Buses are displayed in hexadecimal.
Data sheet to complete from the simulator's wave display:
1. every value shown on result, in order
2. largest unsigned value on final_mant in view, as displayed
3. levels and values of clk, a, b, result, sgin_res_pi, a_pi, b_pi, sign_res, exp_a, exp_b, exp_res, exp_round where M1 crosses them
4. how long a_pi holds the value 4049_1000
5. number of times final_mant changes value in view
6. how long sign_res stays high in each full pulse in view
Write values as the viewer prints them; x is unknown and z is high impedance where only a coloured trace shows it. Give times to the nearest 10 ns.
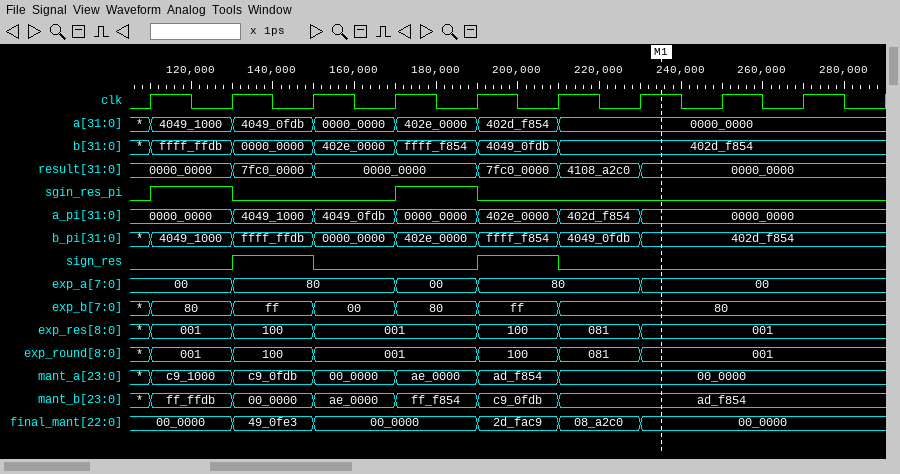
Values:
0000_0000, 7fc0_0000, 0000_0000, 7fc0_0000, 4108_a2c0, 0000_0000
49_0fe3
clk=1, a=0000_0000, b=402d_f854, result=0000_0000, sgin_res_pi=0, a_pi=0000_0000, b_pi=402d_f854, sign_res=0, exp_a=00, exp_b=80, exp_res=001, exp_round=001
20 ns
5
20 ns, 20 ns
